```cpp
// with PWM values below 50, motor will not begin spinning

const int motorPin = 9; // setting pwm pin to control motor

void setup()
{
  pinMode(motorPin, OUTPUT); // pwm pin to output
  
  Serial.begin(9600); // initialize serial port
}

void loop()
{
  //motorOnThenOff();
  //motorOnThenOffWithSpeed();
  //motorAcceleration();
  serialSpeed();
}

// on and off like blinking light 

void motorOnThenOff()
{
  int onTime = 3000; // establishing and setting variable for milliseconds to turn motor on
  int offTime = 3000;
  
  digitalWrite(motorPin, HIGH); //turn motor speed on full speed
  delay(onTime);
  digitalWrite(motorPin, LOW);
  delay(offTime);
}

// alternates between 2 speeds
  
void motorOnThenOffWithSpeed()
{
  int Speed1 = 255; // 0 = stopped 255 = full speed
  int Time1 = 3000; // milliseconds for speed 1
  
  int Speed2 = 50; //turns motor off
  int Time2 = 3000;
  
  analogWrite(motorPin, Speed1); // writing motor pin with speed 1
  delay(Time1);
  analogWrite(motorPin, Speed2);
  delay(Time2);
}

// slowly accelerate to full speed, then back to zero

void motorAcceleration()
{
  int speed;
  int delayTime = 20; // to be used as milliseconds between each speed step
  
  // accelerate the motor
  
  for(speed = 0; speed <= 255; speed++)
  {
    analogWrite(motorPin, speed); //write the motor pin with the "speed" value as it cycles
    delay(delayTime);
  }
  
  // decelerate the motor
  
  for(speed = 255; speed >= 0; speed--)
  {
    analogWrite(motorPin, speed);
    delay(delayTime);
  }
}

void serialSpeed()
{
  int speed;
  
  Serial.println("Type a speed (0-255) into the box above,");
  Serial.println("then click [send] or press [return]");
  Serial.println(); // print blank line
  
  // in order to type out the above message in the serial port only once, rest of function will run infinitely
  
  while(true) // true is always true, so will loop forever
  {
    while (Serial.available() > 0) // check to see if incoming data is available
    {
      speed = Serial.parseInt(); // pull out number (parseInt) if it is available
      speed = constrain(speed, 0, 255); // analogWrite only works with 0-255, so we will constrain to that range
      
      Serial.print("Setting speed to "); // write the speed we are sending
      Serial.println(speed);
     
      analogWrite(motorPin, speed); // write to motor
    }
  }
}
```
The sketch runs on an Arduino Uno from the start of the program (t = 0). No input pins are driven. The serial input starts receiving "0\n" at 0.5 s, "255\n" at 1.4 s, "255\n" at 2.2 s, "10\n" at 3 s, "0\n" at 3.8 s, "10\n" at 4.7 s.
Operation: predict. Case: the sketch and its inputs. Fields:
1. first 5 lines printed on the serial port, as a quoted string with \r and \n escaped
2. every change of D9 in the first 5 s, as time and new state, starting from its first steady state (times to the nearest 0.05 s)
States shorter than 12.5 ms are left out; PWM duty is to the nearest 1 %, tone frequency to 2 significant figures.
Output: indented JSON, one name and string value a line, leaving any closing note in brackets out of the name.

{
  "first 5 lines printed on the serial port, as a quoted string with \\r and \\n escaped": "\"Type a speed (0-255) into the box above,\\r\\nthen click [send] or press [return]\\r\\n\\r\\nSetting speed to 0\\r\\nSetting speed to 255\\r\\n\"",
  "every change of D9 in the first 5 s, as time and new state, starting from its first steady state": "0 s low; 1.4 s high; 3 s PWM 4 %; 3.8 s low; 4.7 s PWM 4 %"
}
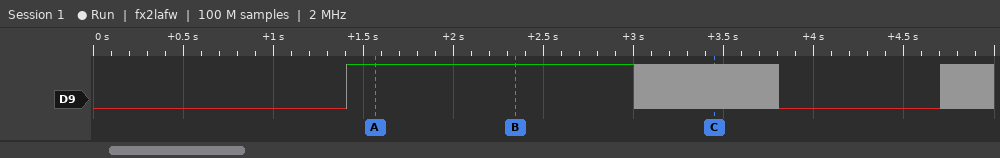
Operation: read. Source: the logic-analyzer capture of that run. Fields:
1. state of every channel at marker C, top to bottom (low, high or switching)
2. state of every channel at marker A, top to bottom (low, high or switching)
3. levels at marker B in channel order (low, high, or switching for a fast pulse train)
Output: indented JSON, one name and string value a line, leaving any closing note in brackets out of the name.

{
  "state of every channel at marker C, top to bottom": "D9 switching",
  "state of every channel at marker A, top to bottom": "D9 high",
  "levels at marker B in channel order": "D9 high"
}
